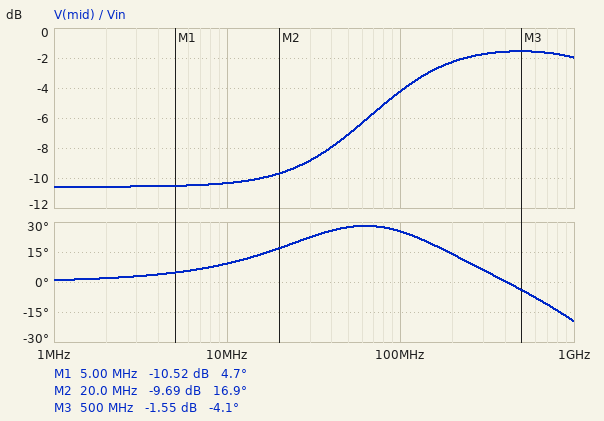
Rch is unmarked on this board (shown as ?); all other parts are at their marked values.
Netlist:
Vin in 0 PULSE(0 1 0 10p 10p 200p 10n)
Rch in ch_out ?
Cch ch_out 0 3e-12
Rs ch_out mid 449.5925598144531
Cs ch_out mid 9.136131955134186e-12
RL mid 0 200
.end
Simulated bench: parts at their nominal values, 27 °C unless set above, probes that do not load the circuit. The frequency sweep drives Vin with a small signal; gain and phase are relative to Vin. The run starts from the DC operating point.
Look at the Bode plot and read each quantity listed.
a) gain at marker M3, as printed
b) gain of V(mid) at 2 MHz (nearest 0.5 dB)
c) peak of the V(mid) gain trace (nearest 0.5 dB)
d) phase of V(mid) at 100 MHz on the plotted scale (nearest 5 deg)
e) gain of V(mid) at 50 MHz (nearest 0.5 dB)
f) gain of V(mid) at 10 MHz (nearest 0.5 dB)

-1.55 dB
-10.5 dB
-1.5 dB
25 deg
-7.0 dB
-10.5 dB
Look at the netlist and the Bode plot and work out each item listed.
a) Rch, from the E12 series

27 Ω
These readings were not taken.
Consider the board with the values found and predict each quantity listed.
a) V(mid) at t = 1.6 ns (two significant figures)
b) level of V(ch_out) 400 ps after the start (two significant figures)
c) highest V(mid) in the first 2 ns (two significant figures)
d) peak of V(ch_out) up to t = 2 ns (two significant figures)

-32 mV
72 mV
770 mV
840 mV
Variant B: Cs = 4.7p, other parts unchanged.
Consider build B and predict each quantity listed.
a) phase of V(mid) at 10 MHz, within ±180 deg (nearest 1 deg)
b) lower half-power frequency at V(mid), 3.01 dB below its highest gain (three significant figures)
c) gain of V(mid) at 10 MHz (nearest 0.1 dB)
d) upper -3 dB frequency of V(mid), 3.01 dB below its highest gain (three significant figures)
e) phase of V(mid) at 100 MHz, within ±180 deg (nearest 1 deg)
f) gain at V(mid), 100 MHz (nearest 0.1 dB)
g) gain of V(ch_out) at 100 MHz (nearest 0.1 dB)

5 deg
162 MHz
-10.5 dB
2.64 GHz
26 deg
-7.0 dB
-0.5 dB
